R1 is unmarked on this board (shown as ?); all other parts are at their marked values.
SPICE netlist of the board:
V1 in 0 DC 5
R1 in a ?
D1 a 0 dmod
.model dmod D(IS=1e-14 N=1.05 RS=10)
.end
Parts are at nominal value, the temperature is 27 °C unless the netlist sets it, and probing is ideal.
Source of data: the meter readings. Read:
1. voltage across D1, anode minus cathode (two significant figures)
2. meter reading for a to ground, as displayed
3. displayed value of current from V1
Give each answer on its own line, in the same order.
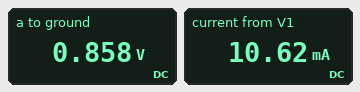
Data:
860 mV
0.858 V
10.62 mA
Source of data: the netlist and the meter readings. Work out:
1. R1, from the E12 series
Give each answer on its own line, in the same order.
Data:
390 Ω
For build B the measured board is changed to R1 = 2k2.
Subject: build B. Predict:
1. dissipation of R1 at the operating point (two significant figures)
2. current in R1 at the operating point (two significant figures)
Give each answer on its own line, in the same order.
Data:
8.3 mW
1.9 mA
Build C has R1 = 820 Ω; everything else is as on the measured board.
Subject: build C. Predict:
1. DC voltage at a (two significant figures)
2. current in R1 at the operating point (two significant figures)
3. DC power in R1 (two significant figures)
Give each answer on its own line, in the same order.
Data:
780 mV
5.1 mA
22 mW
